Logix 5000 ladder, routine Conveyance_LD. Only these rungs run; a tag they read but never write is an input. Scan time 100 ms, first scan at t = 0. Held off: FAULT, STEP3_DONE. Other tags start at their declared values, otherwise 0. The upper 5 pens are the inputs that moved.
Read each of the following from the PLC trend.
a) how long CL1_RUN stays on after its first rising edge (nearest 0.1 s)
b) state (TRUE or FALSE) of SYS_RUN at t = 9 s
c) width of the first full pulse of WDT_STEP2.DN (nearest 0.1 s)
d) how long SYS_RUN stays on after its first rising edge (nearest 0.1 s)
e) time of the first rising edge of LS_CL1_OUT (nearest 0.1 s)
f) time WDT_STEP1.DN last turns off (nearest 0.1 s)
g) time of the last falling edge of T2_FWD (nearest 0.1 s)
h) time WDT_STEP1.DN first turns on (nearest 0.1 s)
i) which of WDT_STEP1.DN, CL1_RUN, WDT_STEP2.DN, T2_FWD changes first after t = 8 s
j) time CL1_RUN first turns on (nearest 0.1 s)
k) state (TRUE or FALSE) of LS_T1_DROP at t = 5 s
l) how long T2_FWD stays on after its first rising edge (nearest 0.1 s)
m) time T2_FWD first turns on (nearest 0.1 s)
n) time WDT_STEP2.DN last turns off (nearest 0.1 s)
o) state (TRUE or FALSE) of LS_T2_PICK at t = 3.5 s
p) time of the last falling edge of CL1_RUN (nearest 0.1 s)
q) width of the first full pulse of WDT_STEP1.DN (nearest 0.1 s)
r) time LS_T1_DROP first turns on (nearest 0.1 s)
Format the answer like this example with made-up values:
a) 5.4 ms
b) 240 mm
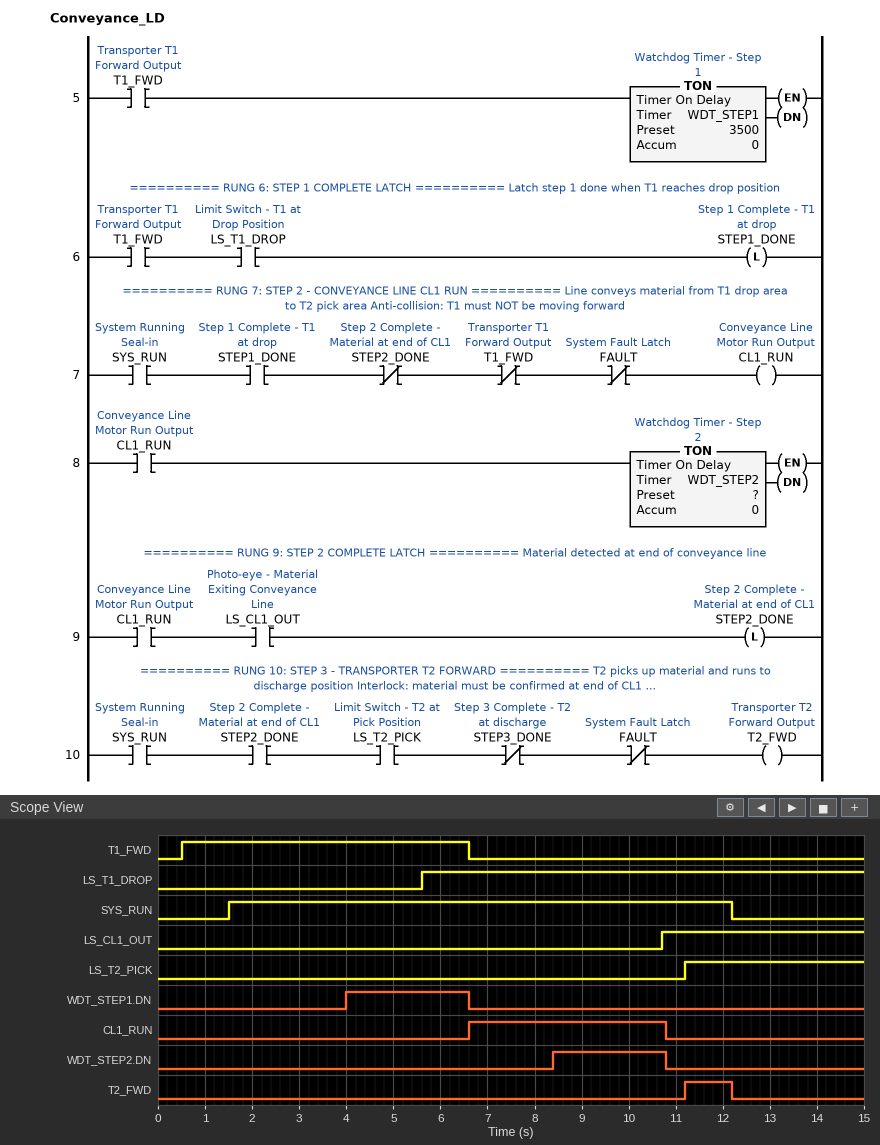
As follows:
a) 4.2 s
b) TRUE
c) 2.4 s
d) 10.7 s
e) 10.7 s
f) 6.6 s
g) 12.2 s
h) 4.0 s
i) WDT_STEP2.DN
j) 6.6 s
k) FALSE
l) 1.0 s
m) 11.2 s
n) 10.8 s
o) FALSE
p) 10.8 s
q) 2.6 s
r) 5.6 s
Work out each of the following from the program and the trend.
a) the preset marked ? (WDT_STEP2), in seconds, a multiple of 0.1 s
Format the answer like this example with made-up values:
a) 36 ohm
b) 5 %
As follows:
a) 1.8 s
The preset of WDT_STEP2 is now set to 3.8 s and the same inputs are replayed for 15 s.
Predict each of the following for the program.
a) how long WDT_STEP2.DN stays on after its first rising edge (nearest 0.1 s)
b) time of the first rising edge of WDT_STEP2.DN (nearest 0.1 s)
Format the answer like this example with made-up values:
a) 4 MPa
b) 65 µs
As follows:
a) 0.4 s
b) 10.4 s
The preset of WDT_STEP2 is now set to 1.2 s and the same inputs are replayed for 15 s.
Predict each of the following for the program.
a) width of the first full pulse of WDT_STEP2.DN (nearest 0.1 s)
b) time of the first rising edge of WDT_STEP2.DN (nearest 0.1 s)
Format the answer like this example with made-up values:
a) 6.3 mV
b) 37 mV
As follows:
a) 3.0 s
b) 7.8 s
